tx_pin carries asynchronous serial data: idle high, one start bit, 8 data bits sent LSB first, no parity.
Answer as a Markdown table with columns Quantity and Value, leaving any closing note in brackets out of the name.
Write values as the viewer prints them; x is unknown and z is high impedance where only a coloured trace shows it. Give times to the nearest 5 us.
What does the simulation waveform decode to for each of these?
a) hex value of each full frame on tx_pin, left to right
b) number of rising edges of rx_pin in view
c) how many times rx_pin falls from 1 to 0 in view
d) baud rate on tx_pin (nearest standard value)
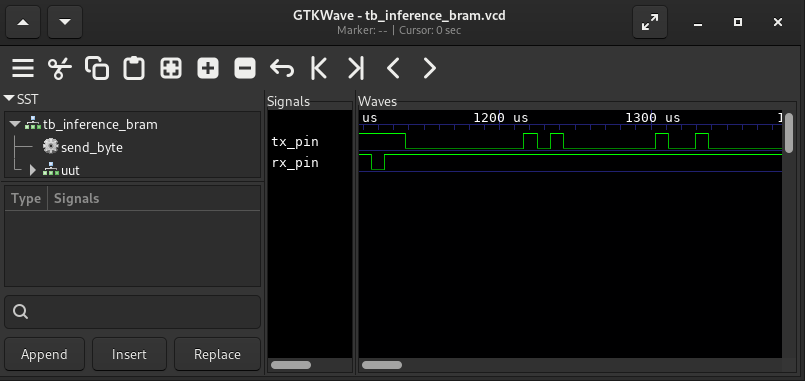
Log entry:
| Quantity | Value |
|---|---|
| hex value of each full frame on tx_pin, left to right | 00, 01 |
| number of rising edges of rx_pin in view | 1 |
| how many times rx_pin falls from 1 to 0 in view | 1 |
| baud rate on tx_pin | 115200 baud |
